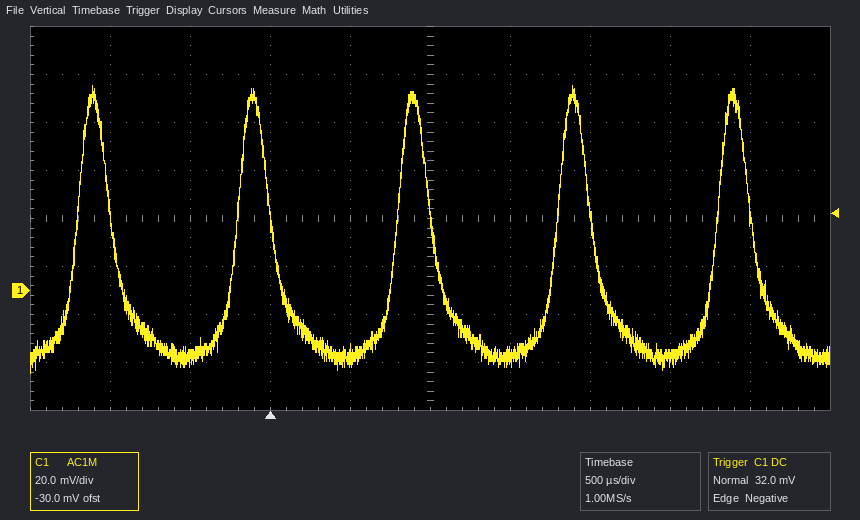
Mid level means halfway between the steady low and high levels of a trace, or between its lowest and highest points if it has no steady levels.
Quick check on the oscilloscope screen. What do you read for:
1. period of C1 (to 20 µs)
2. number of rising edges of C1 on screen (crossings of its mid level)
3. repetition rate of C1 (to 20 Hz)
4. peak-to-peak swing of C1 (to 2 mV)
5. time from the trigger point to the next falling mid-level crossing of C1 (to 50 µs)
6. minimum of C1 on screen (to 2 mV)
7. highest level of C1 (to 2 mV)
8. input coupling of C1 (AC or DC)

1.00 ms
5
1.00 kHz
120 mV
1.00 ms
-34 mV
86 mV
AC
